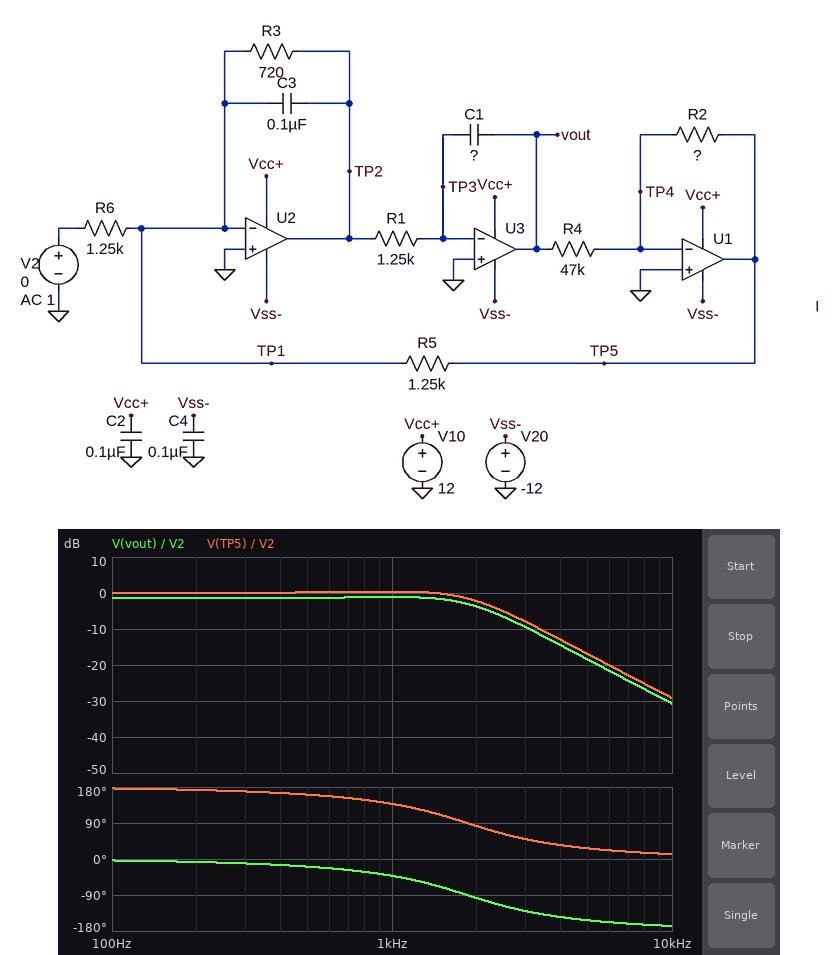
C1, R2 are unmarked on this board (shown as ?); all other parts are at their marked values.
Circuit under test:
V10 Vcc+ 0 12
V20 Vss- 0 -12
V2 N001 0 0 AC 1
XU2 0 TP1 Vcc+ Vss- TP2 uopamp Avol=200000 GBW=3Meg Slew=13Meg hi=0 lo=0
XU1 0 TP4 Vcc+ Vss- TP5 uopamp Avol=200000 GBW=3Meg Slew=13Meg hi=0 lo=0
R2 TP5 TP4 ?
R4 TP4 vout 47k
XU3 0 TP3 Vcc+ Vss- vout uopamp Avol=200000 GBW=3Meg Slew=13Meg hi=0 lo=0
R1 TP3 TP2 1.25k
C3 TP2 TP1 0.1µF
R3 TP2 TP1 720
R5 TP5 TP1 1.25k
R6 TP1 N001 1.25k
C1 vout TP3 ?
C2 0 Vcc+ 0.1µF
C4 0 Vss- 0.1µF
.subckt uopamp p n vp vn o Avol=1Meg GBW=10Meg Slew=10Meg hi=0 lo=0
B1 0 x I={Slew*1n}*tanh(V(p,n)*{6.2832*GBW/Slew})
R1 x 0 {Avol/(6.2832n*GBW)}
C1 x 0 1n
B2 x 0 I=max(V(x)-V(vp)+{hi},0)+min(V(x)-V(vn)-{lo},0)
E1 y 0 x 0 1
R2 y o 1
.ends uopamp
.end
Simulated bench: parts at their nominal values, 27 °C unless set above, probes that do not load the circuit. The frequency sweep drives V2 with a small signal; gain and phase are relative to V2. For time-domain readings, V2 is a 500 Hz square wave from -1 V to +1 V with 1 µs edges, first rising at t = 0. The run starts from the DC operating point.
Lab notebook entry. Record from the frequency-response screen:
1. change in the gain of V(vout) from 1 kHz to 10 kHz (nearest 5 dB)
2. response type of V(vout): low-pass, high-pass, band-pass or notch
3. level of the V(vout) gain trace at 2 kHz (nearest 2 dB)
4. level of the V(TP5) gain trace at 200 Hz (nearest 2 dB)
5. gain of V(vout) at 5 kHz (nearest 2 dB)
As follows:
-30 dB
low-pass
-4 dB
0 dB
-18 dB
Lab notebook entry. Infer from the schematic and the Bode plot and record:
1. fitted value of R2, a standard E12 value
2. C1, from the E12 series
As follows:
56 kΩ
56 nF
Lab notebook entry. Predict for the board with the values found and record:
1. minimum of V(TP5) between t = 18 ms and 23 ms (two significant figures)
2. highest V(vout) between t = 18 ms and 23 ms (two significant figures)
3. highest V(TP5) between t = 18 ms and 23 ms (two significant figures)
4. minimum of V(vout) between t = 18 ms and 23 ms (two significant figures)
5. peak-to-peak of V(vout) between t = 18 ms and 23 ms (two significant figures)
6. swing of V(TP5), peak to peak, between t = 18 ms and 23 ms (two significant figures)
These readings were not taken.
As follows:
-1.2 V
1.0 V
1.2 V
-1.0 V
2.0 V
2.4 V
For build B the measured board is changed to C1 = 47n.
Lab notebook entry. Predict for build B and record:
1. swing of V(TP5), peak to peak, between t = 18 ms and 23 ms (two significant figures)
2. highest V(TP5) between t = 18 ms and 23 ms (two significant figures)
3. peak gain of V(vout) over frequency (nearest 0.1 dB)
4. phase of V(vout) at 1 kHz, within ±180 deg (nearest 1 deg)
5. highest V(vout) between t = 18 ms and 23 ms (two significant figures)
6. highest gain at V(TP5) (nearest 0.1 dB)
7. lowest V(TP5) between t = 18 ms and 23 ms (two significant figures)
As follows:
2.5 V
1.3 V
-0.7 dB
-35 deg
1.1 V
0.8 dB
-1.3 V
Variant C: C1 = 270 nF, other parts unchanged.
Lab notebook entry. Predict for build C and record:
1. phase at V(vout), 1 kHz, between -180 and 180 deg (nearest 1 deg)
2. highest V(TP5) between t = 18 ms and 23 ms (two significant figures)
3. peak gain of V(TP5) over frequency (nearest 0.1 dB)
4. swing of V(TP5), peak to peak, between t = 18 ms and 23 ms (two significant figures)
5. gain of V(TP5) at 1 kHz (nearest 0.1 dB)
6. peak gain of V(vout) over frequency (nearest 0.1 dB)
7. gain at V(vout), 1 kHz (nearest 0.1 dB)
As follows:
-97 deg
800 mV
0 dB
1.6 V
-9.9 dB
-1.5 dB
-11.4 dB
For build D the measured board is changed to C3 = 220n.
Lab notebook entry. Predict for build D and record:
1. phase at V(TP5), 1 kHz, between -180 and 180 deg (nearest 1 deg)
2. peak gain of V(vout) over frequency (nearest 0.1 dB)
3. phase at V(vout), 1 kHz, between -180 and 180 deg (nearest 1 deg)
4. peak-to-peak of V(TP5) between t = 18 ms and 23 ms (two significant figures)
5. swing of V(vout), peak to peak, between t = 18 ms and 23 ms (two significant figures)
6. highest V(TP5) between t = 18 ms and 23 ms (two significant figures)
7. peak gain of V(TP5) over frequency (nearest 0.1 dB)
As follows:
119 deg
1.2 dB
-61 deg
3.0 V
2.5 V
1.5 V
2.7 dB
